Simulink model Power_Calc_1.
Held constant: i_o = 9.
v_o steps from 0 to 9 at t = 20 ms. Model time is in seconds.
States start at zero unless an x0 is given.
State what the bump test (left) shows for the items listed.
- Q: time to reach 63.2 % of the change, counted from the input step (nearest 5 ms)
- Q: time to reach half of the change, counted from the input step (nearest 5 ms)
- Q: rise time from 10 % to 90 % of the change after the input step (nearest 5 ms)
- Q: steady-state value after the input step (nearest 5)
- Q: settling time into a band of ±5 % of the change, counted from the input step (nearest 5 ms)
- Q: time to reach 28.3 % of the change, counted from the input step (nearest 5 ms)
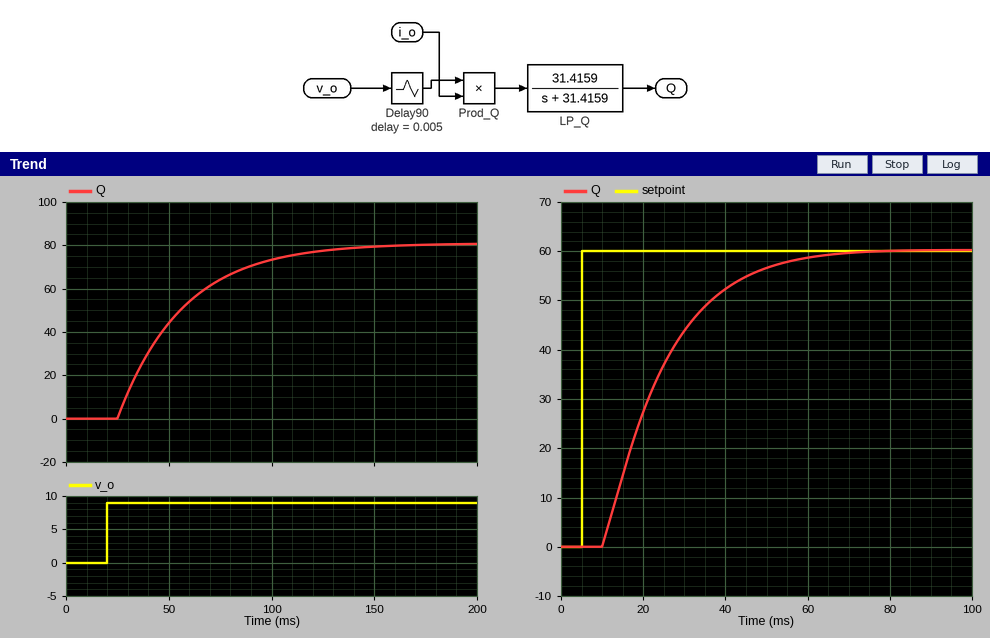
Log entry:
35 ms
25 ms
70 ms
80
100 ms
15 ms
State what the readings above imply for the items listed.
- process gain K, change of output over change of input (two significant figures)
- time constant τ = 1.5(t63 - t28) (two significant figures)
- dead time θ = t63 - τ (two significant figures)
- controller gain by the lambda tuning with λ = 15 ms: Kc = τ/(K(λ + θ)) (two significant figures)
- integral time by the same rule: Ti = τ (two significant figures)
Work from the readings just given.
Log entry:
8.9
30 ms
5.0 ms
0.17
30 ms
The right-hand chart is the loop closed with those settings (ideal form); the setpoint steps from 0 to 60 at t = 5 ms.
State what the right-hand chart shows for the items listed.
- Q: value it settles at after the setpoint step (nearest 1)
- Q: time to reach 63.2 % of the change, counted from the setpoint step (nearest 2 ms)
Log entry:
60
20 ms
